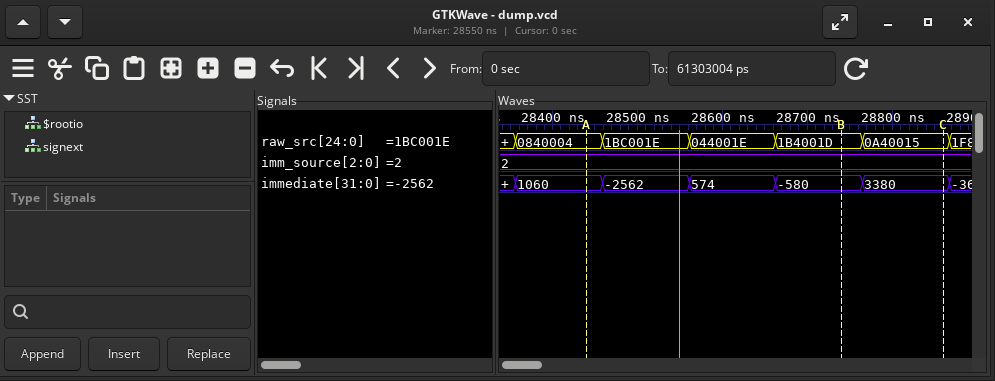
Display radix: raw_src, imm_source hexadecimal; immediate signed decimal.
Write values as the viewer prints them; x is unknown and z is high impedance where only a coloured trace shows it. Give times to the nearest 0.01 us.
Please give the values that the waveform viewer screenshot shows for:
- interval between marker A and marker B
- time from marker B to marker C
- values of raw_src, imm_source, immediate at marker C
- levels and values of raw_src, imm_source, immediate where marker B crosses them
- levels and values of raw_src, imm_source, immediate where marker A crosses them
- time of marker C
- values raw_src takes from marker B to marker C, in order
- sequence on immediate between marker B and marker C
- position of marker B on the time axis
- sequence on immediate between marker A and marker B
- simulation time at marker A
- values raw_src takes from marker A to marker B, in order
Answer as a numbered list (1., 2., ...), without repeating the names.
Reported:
1. 0.3 us
2. 0.12 us
3. raw_src=0A40015, imm_source=2, immediate=3380
4. raw_src=1B4001D, imm_source=2, immediate=-580
5. raw_src=0840004, imm_source=2, immediate=1060
6. 28.86 us
7. 1B4001D, 0A40015
8. -580, 3380
9. 28.74 us
10. 1060, -2562, 574, -580
11. 28.44 us
12. 0840004, 1BC001E, 044001E, 1B4001D
